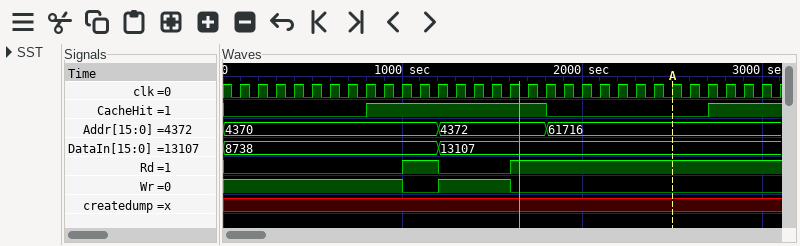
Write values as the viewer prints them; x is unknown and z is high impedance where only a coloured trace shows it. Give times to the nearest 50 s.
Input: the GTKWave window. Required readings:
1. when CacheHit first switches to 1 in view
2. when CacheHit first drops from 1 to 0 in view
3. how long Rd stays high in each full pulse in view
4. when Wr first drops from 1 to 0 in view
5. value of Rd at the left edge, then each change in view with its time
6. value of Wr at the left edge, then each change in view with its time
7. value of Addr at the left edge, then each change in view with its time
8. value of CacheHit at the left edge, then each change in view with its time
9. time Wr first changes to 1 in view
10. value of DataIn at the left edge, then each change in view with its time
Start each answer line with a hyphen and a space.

- 800 s
- 1800 s
- 200 s
- 1000 s
- 0, 1 at 1000 s, 0 at 1200 s, 1 at 1600 s
- 1, 0 at 1000 s, 1 at 1200 s, 0 at 1600 s
- 4370, 4372 at 1200 s, 61716 at 1800 s
- 0, 1 at 800 s, 0 at 1800 s, 1 at 2700 s
- 1200 s
- 8738, 13107 at 1200 s
